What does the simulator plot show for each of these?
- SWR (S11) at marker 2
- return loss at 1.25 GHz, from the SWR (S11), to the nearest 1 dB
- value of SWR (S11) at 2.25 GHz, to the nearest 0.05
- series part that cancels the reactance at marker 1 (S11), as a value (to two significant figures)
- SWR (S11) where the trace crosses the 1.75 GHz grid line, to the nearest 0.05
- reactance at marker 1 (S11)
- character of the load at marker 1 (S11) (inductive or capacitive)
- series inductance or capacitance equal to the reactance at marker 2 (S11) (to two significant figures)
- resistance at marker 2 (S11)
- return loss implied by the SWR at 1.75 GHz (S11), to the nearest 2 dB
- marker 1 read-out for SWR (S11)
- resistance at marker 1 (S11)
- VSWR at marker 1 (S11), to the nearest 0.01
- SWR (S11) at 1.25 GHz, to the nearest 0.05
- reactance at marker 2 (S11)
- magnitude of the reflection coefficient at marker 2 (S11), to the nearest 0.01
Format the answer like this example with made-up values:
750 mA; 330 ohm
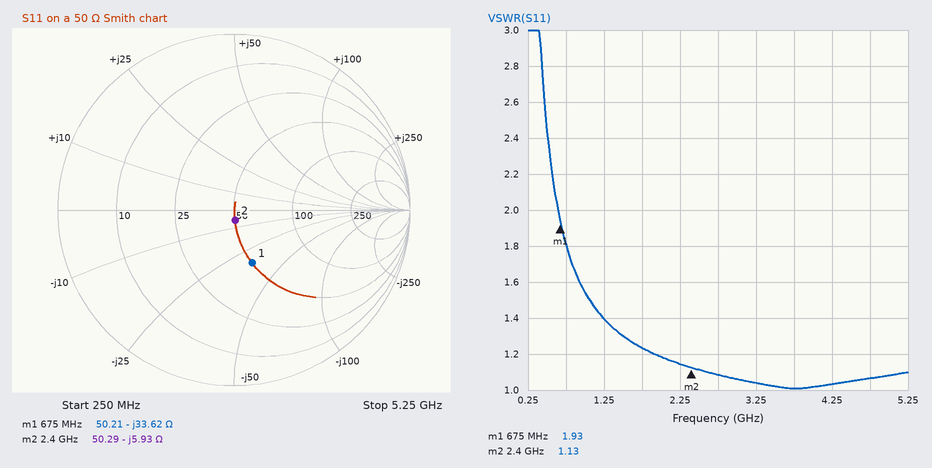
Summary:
1.13; 16 dB; 1.15; 7.9 nH; 1.25; -33.62 Ω; capacitive; 11 pF; 50.29 Ω; 20 dB; 1.93; 50.21 Ω; 1.93; 1.40; -5.93 Ω; 0.06
